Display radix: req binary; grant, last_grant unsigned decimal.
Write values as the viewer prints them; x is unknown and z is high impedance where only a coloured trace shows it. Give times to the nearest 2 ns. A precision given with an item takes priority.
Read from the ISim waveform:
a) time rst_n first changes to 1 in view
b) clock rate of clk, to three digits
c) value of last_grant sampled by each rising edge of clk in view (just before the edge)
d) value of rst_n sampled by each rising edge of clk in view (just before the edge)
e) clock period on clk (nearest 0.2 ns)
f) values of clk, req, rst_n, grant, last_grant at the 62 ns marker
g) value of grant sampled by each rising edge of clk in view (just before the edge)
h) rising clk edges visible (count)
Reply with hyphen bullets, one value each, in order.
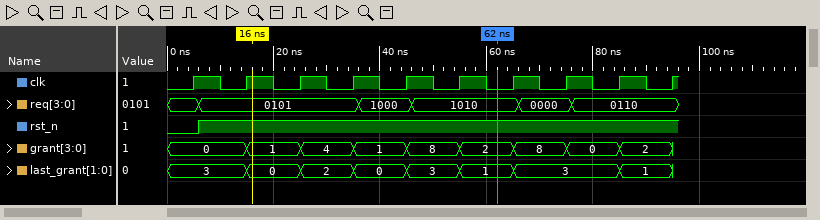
- 6 ns
- 100 MHz
- 3, 3, 0, 2, 0, 3, 1, 3, 3, 1
- 0 1 1 1 1 1 1 1 1 1
- 10 ns
- clk=0, req=1010, rst_n=1, grant=2, last_grant=1
- 0, 0, 1, 4, 1, 8, 2, 8, 0, 2
- 10
